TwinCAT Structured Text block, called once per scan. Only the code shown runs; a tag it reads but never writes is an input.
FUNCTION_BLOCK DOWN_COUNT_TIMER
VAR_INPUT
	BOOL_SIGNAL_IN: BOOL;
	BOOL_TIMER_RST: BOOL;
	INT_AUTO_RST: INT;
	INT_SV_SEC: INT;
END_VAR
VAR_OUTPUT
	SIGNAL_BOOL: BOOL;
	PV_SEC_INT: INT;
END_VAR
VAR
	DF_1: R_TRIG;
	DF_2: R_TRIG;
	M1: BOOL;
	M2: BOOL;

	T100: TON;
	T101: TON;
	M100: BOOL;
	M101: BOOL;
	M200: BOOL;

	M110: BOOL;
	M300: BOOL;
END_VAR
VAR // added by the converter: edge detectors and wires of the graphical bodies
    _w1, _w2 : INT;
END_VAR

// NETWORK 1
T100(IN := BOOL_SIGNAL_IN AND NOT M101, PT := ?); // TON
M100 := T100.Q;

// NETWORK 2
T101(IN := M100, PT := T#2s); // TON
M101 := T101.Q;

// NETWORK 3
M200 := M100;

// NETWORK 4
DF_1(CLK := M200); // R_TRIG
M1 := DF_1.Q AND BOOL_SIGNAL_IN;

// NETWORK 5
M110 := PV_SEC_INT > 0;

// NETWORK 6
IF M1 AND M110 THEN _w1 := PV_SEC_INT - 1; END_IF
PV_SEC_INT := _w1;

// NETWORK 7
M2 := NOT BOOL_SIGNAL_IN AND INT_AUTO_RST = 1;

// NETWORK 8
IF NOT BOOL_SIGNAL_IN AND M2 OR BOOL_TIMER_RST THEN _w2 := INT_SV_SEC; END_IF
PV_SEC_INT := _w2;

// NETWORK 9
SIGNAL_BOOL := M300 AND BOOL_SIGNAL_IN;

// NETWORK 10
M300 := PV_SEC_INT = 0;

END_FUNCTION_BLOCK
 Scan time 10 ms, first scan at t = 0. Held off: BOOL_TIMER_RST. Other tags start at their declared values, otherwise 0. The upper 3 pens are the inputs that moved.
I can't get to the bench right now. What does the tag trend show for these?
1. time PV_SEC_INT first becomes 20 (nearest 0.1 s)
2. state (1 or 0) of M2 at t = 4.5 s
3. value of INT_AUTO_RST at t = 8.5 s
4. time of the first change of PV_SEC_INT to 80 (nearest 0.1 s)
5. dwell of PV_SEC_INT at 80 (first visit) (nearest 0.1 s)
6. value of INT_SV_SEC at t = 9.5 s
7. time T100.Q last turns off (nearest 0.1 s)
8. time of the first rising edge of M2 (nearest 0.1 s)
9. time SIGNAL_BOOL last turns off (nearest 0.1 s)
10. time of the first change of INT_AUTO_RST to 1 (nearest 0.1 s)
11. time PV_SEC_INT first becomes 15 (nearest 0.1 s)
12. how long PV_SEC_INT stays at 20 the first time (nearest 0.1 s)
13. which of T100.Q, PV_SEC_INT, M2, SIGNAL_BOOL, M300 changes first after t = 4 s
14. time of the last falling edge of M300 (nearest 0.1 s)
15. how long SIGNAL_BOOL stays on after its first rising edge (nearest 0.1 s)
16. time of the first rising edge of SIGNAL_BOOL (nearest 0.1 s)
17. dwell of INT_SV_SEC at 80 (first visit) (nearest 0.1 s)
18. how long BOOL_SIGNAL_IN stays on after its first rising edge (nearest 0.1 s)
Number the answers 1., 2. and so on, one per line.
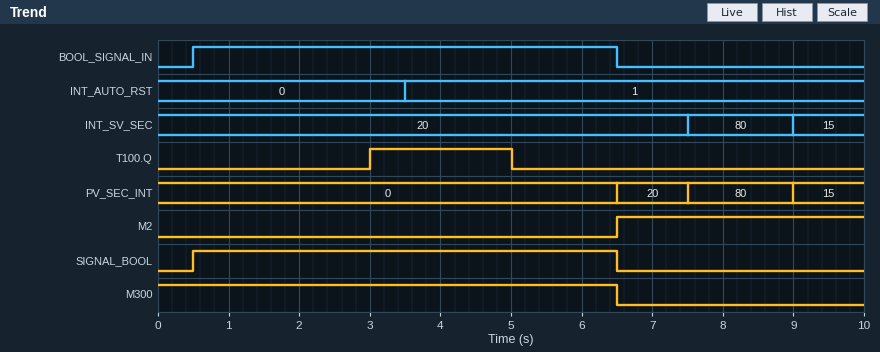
1. 6.5 s
2. 0
3. 1
4. 7.5 s
5. 1.5 s
6. 15
7. 5.0 s
8. 6.5 s
9. 6.5 s
10. 3.5 s
11. 9.0 s
12. 1.0 s
13. T100.Q
14. 6.5 s
15. 6.0 s
16. 0.5 s
17. 1.5 s
18. 6.0 s
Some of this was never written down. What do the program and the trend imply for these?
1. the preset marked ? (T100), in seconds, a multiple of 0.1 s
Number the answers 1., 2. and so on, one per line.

1. 2.5 s
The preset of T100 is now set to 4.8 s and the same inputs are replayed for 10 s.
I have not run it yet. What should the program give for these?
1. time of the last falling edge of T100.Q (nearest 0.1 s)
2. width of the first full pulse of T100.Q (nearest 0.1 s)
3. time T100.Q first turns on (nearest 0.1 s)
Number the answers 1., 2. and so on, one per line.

1. 6.5 s
2. 1.2 s
3. 5.3 s
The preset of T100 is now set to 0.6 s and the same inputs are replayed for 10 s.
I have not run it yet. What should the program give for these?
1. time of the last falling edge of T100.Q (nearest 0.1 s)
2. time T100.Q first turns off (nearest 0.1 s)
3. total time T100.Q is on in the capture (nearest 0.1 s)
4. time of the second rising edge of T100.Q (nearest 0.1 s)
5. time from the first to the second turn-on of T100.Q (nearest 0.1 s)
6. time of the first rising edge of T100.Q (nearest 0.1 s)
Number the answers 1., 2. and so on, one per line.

1. 6.5 s
2. 3.1 s
3. 4.2 s
4. 3.7 s
5. 2.6 s
6. 1.1 s
